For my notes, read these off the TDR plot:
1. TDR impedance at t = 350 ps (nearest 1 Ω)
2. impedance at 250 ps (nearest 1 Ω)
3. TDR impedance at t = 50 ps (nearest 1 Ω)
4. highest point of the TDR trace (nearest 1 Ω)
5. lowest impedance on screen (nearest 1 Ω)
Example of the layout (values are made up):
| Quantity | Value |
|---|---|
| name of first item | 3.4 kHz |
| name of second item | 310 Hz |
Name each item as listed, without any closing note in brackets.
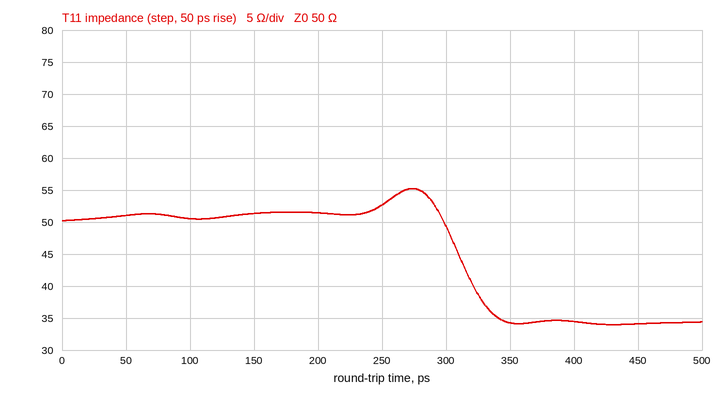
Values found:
| Quantity | Value |
|---|---|
| TDR impedance at t = 350 ps | 34 Ω |
| impedance at 250 ps | 53 Ω |
| TDR impedance at t = 50 ps | 51 Ω |
| highest point of the TDR trace | 55 Ω |
| lowest impedance on screen | 34 Ω |
